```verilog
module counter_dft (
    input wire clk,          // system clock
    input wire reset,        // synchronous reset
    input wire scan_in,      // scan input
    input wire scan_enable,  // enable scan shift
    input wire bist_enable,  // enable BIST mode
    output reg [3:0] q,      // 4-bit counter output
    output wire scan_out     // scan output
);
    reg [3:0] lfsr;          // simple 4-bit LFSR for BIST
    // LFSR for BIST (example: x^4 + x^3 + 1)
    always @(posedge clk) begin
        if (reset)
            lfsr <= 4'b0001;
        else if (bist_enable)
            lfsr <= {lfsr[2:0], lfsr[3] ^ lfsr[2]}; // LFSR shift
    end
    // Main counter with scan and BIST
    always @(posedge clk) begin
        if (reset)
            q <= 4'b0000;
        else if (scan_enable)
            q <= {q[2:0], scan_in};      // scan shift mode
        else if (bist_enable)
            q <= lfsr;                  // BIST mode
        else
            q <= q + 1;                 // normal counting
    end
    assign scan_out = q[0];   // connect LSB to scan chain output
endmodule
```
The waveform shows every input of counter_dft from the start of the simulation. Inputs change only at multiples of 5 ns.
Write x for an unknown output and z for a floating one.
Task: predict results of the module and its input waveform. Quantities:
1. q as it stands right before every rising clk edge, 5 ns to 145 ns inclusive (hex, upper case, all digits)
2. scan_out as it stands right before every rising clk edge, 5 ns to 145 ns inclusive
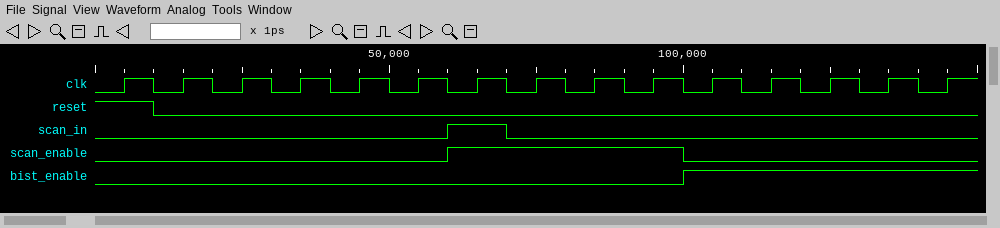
x, 0, 1, 2, 3, 4, 5, B, 6, C, 8, 1, 2, 4, 9
x 0 1 0 1 0 1 1 0 0 0 1 0 0 1
